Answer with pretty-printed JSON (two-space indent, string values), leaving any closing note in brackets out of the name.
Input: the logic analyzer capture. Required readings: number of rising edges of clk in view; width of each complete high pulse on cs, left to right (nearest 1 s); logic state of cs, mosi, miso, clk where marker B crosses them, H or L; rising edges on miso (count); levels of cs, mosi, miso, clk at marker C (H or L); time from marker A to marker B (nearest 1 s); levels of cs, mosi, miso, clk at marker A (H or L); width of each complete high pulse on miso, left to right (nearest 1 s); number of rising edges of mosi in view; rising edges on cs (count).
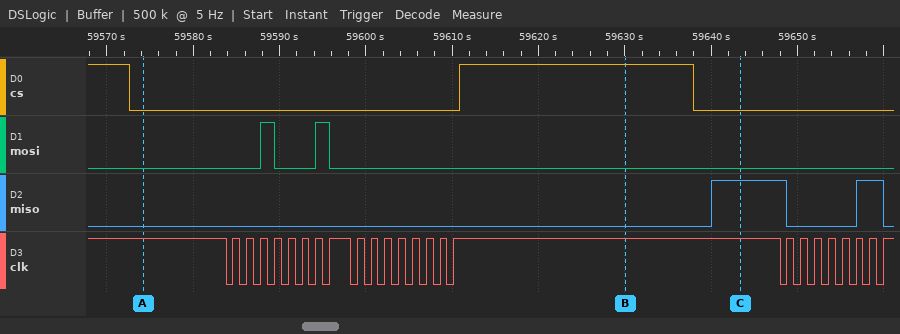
{
  "number of rising edges of clk in view": "24",
  "width of each complete high pulse on cs, left to right": "27 s",
  "logic state of cs, mosi, miso, clk where marker B crosses them, H or L": "cs=H, mosi=L, miso=L, clk=H",
  "rising edges on miso": "2",
  "levels of cs, mosi, miso, clk at marker C": "cs=L, mosi=L, miso=H, clk=H",
  "time from marker A to marker B": "56 s",
  "levels of cs, mosi, miso, clk at marker A": "cs=L, mosi=L, miso=L, clk=H",
  "width of each complete high pulse on miso, left to right": "9 s, 3 s",
  "number of rising edges of mosi in view": "2",
  "rising edges on cs": "1"
}
